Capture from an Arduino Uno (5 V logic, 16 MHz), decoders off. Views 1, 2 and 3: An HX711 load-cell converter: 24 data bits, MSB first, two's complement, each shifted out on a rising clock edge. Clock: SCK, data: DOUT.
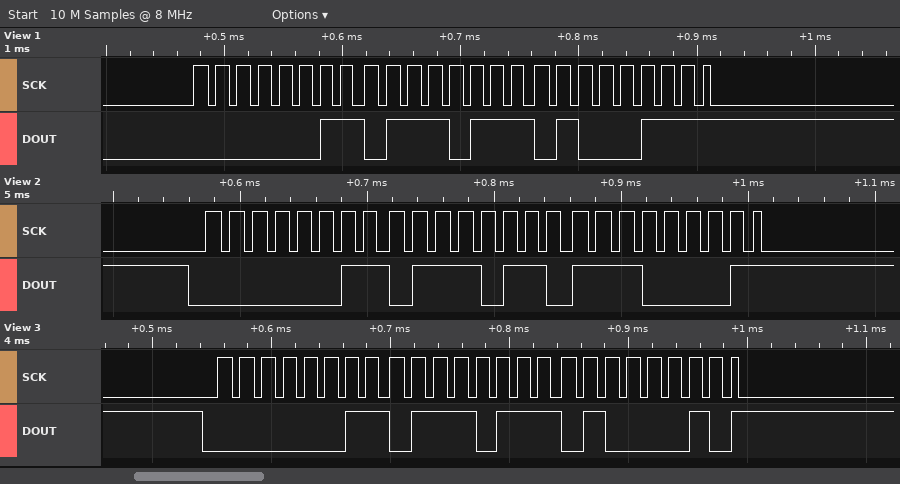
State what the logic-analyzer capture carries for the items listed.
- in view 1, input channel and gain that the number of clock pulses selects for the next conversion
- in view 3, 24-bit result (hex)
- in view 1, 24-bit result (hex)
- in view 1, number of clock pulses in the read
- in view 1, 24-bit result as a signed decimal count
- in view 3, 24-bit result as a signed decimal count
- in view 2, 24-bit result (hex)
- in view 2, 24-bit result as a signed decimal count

channel A, gain 128
0x037742
0x037747
25
227143
227138
0x0376E1
227041
